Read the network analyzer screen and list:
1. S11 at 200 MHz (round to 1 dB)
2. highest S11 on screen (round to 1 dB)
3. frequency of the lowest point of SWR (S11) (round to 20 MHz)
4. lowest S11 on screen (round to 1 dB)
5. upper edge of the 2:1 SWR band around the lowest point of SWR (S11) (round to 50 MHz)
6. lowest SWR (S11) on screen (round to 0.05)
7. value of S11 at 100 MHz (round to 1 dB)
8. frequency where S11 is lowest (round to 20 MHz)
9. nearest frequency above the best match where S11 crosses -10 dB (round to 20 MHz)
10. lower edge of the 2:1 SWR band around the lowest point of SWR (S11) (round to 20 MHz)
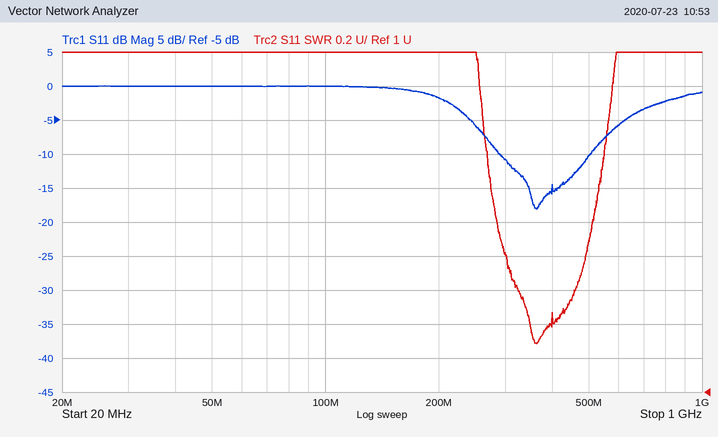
-2 dB
0 dB
360 MHz
-18 dB
500 MHz
1.30
0 dB
360 MHz
500 MHz
280 MHz
